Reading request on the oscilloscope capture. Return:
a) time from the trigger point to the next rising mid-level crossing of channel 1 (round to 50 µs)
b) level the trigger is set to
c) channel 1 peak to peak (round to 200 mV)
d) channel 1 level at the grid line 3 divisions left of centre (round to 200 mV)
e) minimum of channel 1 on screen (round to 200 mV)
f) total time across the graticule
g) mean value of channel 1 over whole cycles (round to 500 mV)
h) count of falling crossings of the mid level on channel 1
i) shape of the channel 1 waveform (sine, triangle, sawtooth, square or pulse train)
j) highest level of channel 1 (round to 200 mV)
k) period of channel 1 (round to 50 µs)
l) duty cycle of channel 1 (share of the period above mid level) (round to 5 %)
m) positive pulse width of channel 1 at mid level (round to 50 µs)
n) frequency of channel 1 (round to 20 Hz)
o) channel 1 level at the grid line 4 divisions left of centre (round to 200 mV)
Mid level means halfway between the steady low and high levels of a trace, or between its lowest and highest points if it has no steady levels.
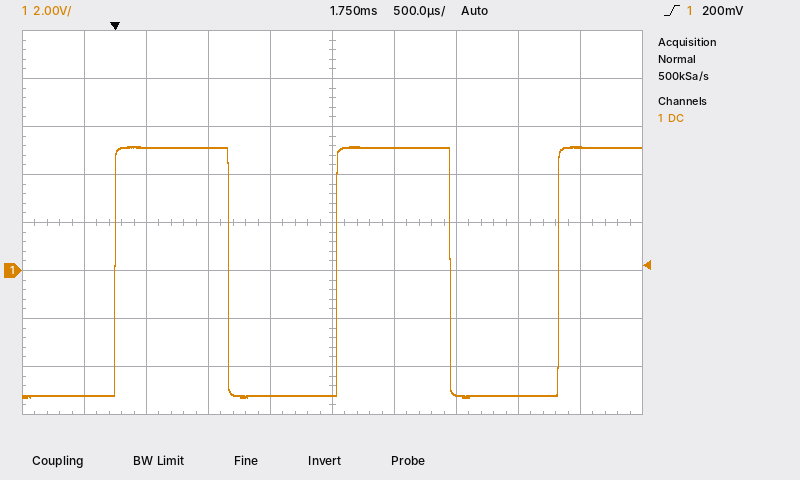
1.80 ms
200 mV
10.4 V
5.2 V
-5.2 V
5 ms
0.0 V
2
square
5.2 V
1.80 ms
50 %
900 µs
560 Hz
-5.2 V
